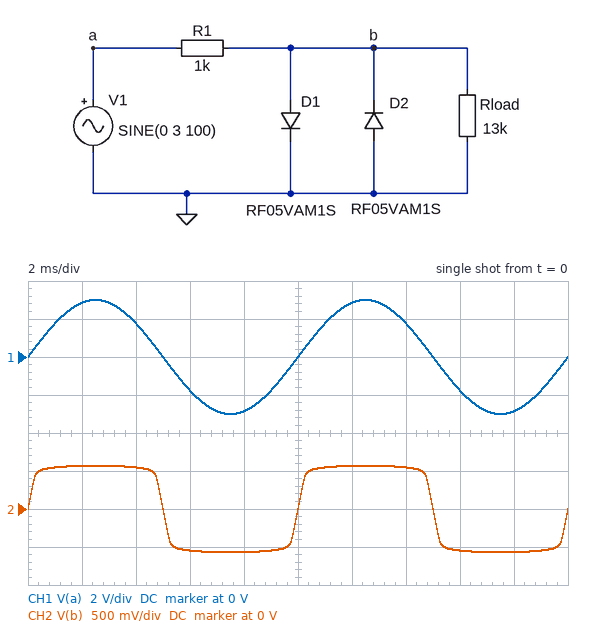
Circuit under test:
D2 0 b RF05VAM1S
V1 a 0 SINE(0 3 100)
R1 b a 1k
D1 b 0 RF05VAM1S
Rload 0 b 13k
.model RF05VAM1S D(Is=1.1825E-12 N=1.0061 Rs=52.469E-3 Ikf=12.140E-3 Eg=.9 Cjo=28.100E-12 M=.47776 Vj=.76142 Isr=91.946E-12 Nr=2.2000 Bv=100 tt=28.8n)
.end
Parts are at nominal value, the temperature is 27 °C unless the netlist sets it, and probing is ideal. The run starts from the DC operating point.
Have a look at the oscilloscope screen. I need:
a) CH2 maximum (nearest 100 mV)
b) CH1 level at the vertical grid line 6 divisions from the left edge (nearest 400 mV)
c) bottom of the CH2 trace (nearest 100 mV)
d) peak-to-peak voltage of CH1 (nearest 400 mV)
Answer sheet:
600 mV
2.8 V
-600 mV
6.0 V
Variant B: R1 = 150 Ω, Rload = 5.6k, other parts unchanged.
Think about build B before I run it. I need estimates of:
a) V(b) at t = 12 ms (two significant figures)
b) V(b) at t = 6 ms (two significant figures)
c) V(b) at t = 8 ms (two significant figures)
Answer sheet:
630 mV
-610 mV
-630 mV
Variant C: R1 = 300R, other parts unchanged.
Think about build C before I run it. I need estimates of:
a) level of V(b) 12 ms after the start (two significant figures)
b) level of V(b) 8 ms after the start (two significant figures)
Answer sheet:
610 mV
-610 mV
